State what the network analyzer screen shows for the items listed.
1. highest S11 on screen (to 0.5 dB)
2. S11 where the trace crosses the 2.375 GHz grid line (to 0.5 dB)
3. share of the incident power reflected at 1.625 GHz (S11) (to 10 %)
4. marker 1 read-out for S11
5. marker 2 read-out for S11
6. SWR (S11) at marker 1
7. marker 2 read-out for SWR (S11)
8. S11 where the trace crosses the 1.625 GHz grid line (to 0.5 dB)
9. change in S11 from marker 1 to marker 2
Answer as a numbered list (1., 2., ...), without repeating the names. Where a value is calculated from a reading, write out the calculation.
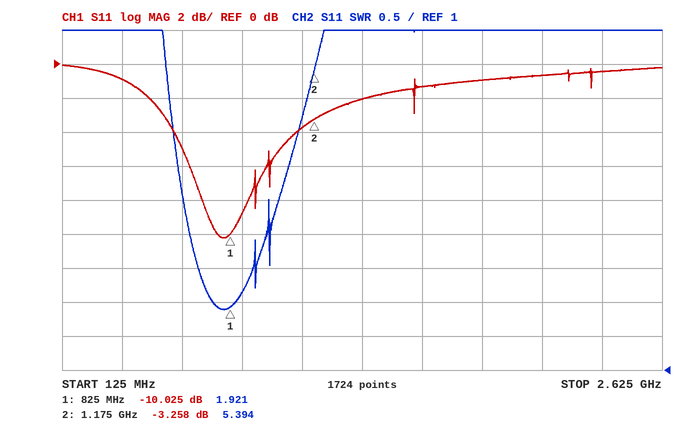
1. 0.0 dB
2. -0.5 dB
3. 10^(-1.5/10) ≈ 70.8 %, so 70 % to the nearest 10 %
4. -10.025 dB
5. -3.258 dB
6. 1.921
7. 5.394
8. -1.5 dB
9. -3.258 − (-10.025) = 6.767 dB
